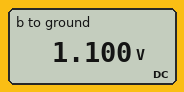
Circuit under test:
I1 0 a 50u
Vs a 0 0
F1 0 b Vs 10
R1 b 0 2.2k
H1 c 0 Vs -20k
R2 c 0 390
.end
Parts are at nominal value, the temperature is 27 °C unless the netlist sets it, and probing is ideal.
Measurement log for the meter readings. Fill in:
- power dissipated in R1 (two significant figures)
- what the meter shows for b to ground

550 µW
1.100 V
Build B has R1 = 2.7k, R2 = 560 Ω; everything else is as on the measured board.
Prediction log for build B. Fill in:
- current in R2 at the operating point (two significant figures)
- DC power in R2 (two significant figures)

1.8 mA
1.8 mW
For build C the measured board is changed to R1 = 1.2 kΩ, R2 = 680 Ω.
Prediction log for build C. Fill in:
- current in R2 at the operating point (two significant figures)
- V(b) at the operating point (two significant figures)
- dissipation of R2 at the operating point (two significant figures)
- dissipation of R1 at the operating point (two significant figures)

1.5 mA
600 mV
1.5 mW
300 µW
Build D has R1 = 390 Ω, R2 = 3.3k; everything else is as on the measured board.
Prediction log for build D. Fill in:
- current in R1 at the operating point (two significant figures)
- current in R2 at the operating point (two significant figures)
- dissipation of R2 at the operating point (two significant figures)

500 µA
300 µA
300 µW
